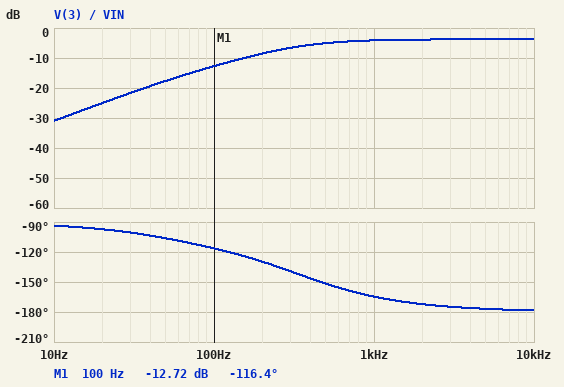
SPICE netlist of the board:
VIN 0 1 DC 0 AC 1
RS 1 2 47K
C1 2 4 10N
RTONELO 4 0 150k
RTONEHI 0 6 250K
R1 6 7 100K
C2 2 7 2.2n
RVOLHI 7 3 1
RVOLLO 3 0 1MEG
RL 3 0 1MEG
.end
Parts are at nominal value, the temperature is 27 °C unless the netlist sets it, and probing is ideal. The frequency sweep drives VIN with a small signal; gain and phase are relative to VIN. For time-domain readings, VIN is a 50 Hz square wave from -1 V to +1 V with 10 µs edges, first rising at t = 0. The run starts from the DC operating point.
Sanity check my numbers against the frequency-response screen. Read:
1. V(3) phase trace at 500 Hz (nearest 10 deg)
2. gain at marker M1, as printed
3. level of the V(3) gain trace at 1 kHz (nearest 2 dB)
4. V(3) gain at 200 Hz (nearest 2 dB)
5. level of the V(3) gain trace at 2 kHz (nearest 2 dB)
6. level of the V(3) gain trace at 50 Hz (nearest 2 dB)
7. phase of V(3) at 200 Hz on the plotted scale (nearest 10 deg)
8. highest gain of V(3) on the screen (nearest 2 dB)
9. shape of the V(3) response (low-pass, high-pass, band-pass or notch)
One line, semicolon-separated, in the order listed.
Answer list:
-150 deg; -12.72 dB; -4 dB; -8 dB; -4 dB; -18 dB; -130 deg; -4 dB; high-pass
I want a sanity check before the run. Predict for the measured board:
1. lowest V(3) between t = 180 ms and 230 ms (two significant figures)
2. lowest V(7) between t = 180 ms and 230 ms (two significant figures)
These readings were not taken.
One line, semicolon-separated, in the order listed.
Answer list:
-1.3 V; -1.3 V
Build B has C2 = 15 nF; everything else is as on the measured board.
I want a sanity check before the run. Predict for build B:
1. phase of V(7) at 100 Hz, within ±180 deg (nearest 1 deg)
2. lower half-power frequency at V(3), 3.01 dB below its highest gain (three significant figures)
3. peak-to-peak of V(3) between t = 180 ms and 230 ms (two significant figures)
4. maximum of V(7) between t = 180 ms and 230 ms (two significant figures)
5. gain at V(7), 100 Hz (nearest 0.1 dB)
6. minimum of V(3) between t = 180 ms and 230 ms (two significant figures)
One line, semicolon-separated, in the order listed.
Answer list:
-163 deg; 31.0 Hz; 2.3 V; 1.2 V; -3.6 dB; -1.2 V
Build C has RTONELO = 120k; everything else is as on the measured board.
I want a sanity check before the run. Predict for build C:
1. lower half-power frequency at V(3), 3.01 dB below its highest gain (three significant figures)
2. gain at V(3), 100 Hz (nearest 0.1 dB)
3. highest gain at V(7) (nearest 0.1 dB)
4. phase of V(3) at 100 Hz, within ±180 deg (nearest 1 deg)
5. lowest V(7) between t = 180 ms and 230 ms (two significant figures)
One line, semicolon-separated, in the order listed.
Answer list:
282 Hz; -12.7 dB; -4.2 dB; -118 deg; -1.2 V
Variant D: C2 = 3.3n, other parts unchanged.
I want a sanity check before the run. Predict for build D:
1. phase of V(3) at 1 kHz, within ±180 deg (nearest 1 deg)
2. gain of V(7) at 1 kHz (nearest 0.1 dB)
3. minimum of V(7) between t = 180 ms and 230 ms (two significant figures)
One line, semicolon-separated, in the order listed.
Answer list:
-170 deg; -3.9 dB; -1.3 V
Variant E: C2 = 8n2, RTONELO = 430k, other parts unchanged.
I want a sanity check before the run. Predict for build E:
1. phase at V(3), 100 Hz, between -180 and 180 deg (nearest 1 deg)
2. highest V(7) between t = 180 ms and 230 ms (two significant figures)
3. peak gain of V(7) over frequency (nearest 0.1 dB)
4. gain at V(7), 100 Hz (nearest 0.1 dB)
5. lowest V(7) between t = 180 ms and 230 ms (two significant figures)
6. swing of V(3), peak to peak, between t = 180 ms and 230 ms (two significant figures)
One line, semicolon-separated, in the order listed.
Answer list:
-144 deg; 1.5 V; -2.5 dB; -4.5 dB; -1.5 V; 2.9 V
